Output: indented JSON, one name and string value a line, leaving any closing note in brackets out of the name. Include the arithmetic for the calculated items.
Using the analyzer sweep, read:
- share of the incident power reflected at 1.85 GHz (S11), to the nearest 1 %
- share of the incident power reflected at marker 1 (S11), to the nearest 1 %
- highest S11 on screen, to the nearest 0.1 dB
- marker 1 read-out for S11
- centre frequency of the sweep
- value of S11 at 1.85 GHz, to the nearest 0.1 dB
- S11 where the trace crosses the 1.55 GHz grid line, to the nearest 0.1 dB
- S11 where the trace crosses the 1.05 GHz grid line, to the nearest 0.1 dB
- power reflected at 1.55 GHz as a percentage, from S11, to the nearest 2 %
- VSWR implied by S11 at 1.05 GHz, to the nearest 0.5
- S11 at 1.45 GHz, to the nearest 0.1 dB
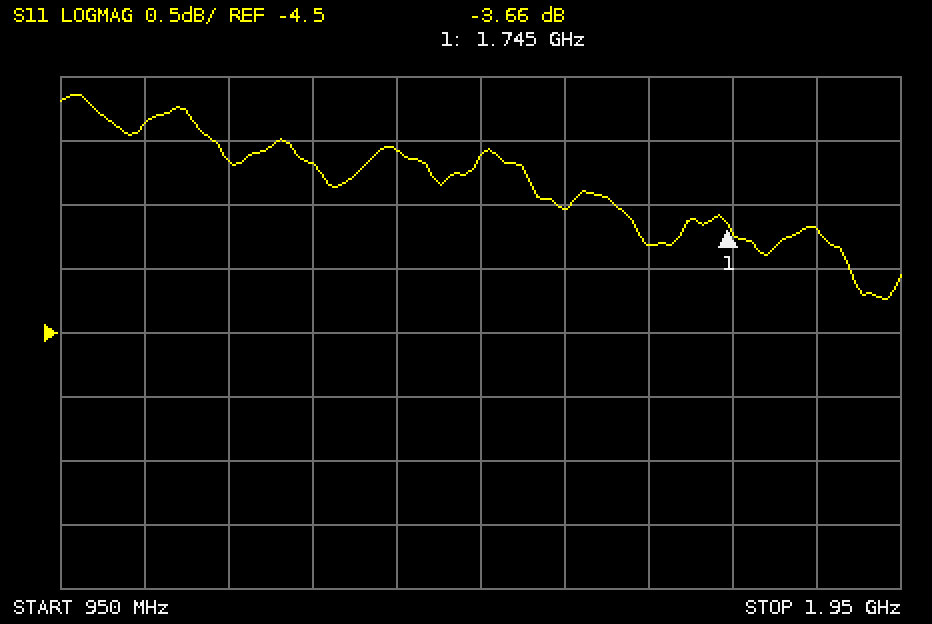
{
  "share of the incident power reflected at 1.85 GHz (S11), to the nearest 1 %": "10^(-3.7/10) ≈ 43 %",
  "share of the incident power reflected at marker 1 (S11), to the nearest 1 %": "10^(-3.66/10) ≈ 43 %",
  "highest S11 on screen, to the nearest 0.1 dB": "-2.6 dB",
  "marker 1 read-out for S11": "-3.66 dB",
  "centre frequency of the sweep": "1.45 GHz",
  "value of S11 at 1.85 GHz, to the nearest 0.1 dB": "-3.7 dB",
  "S11 where the trace crosses the 1.55 GHz grid line, to the nearest 0.1 dB": "-3.5 dB",
  "S11 where the trace crosses the 1.05 GHz grid line, to the nearest 0.1 dB": "-2.9 dB",
  "power reflected at 1.55 GHz as a percentage, from S11, to the nearest 2 %": "10^(-3.5/10) ≈ 44.7 %, so 44 % to the nearest 2 %",
  "VSWR implied by S11 at 1.05 GHz, to the nearest 0.5": "|Γ| = 10^(-2.9/20) = 0.7161; VSWR = (1 + 0.7161)/(1 − 0.7161) ≈ 6.0",
  "S11 at 1.45 GHz, to the nearest 0.1 dB": "-3.1 dB"
}
